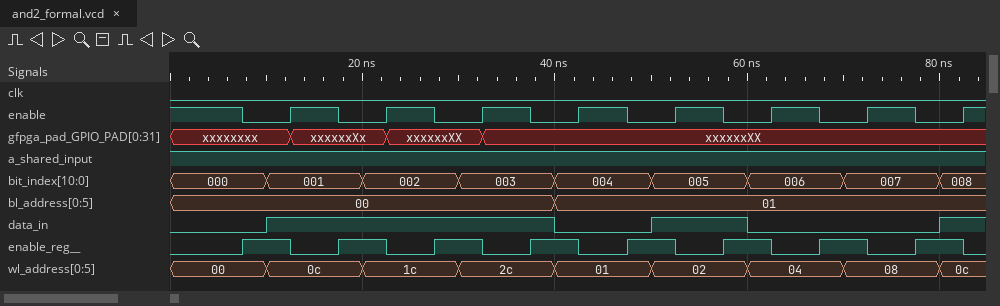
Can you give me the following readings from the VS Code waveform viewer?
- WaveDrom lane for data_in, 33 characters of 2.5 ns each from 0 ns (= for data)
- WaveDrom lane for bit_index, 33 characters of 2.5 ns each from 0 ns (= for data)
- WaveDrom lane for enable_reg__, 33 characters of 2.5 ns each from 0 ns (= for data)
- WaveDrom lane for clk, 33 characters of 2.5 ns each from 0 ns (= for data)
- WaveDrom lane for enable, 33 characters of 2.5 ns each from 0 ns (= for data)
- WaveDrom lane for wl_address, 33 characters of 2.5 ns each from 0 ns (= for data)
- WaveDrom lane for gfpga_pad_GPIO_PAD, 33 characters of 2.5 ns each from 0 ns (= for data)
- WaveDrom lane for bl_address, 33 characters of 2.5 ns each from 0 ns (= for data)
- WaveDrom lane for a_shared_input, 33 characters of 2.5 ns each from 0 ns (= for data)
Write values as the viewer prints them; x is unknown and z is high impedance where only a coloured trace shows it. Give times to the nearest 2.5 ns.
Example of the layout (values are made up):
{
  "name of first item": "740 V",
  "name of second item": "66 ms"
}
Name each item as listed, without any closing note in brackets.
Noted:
{
  "WaveDrom lane for data_in, 33 characters of 2.5 ns each from 0 ns": "{name: 'data_in', wave: '0...1...........0...1...0.......1'}",
  "WaveDrom lane for bit_index, 33 characters of 2.5 ns each from 0 ns": "{name: 'bit_index', wave: '=...=...=...=...=...=...=...=...=', data: '000 001 002 003 004 005 006 007 008'}",
  "WaveDrom lane for enable_reg__, 33 characters of 2.5 ns each from 0 ns": "{name: 'enable_reg__', wave: '0..1.0.1.0.1.0.1.0.1.0.1.0.1.0.1.'}",
  "WaveDrom lane for clk, 33 characters of 2.5 ns each from 0 ns": "{name: 'clk', wave: '0................................'}",
  "WaveDrom lane for enable, 33 characters of 2.5 ns each from 0 ns": "{name: 'enable', wave: '1..0.1.0.1.0.1.0.1.0.1.0.1.0.1.0.'}",
  "WaveDrom lane for wl_address, 33 characters of 2.5 ns each from 0 ns": "{name: 'wl_address', wave: '=...=...=...=...=...=...=...=...=', data: '00 0c 1c 2c 01 02 04 08 0c'}",
  "WaveDrom lane for gfpga_pad_GPIO_PAD, 33 characters of 2.5 ns each from 0 ns": "{name: 'gfpga_pad_GPIO_PAD', wave: 'x....=...=...=...................', data: 'xxxxxxXx xxxxxxXX xxxxxxXX'}",
  "WaveDrom lane for bl_address, 33 characters of 2.5 ns each from 0 ns": "{name: 'bl_address', wave: '=...............=................', data: '00 01'}",
  "WaveDrom lane for a_shared_input, 33 characters of 2.5 ns each from 0 ns": "{name: 'a_shared_input', wave: '1................................'}"
}
